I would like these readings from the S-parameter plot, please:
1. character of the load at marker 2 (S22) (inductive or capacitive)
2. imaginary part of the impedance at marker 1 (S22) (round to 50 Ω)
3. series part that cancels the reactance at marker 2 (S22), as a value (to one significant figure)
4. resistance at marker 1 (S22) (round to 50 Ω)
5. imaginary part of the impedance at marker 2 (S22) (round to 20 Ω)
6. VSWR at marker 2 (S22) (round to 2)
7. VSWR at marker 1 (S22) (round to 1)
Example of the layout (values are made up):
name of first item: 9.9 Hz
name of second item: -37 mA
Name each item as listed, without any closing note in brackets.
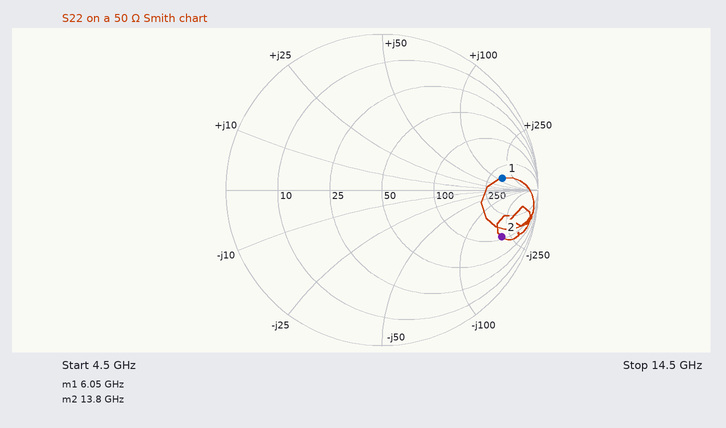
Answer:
character of the load at marker 2 (S22): capacitive
imaginary part of the impedance at marker 1 (S22): +150 Ω
series part that cancels the reactance at marker 2 (S22), as a value: 2 nH
resistance at marker 1 (S22): 350 Ω
imaginary part of the impedance at marker 2 (S22): -200 Ω
VSWR at marker 2 (S22): 10
VSWR at marker 1 (S22): 8
